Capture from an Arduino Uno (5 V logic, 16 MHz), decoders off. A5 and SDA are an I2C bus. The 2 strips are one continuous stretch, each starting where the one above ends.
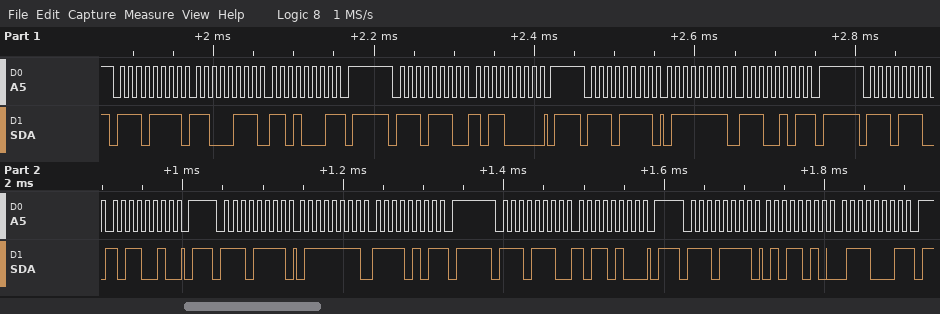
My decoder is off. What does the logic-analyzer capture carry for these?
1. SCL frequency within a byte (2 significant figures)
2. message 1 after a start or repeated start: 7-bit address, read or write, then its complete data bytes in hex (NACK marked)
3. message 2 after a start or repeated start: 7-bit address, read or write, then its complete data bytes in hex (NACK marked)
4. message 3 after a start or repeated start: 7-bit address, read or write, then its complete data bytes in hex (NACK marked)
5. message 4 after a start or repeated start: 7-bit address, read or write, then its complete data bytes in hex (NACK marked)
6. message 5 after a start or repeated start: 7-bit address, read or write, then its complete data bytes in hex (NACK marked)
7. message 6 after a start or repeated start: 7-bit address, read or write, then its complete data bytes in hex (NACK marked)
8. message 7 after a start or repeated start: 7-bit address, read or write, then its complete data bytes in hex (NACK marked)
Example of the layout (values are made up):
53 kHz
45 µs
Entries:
100 kHz
0x77 read: C7 D1 NACK
0x77 write: B0
0x77 read: 7F E5 NACK
0x77 write: B2
0x77 read: 7F F5 NACK
0x77 write: B4
0x77 read: 5A 71 NACK
